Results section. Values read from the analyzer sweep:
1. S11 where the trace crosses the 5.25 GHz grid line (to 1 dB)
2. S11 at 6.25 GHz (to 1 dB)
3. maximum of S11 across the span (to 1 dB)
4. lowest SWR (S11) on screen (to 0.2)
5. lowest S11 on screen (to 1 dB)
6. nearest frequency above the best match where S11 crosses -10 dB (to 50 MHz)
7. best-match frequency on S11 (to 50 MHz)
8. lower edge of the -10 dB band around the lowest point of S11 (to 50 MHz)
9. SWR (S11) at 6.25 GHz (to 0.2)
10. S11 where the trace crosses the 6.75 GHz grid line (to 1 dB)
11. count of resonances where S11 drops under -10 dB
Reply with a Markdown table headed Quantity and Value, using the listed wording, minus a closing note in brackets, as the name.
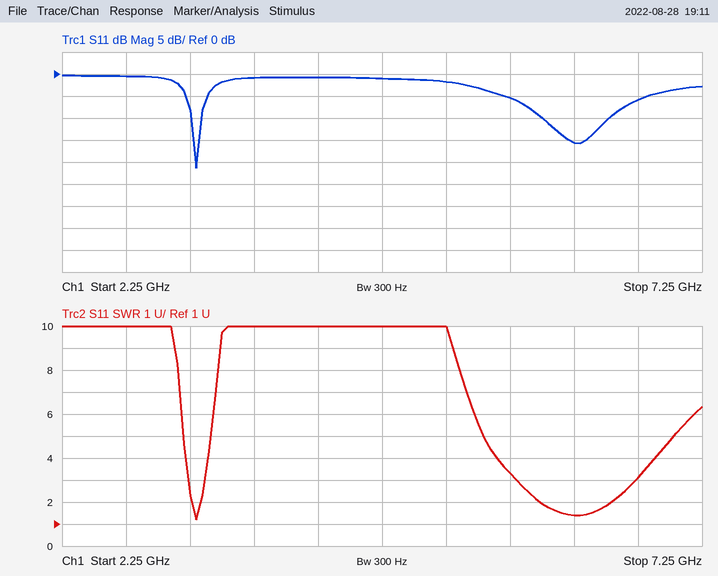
| Quantity | Value |
|---|---|
| S11 where the trace crosses the 5.25 GHz grid line | -2 dB |
| S11 at 6.25 GHz | -16 dB |
| maximum of S11 across the span | 0 dB |
| lowest SWR (S11) on screen | 1.2 |
| lowest S11 on screen | -21 dB |
| nearest frequency above the best match where S11 crosses -10 dB | 3.35 GHz |
| best-match frequency on S11 | 3.30 GHz |
| lower edge of the -10 dB band around the lowest point of S11 | 3.25 GHz |
| SWR (S11) at 6.25 GHz | 1.4 |
| S11 where the trace crosses the 6.75 GHz grid line | -6 dB |
| count of resonances where S11 drops under -10 dB | 2 |
